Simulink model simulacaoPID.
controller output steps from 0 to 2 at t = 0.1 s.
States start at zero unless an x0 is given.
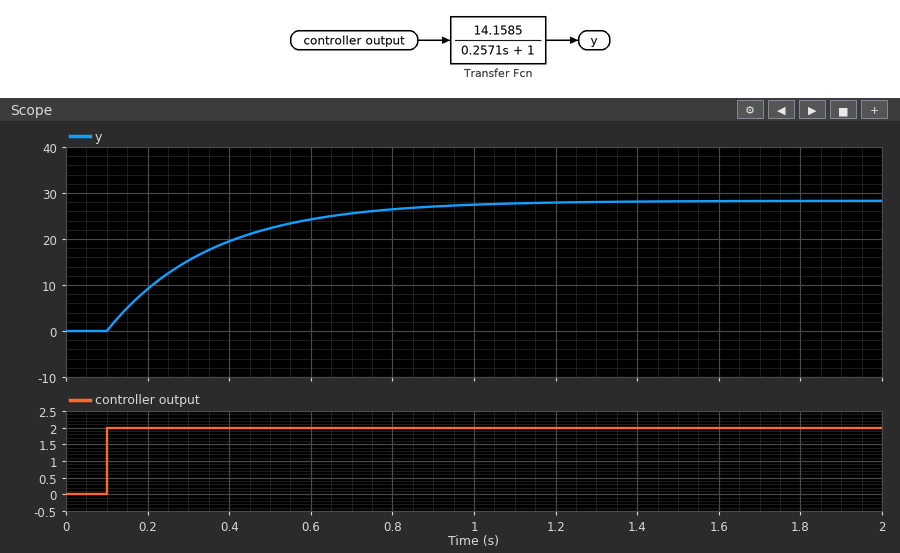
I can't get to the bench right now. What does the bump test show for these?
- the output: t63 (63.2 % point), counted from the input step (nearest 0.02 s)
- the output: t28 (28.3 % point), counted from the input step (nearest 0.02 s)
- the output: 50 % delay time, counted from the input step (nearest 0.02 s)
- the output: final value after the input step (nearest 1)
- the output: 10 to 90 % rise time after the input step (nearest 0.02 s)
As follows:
0.26 s
0.08 s
0.18 s
28
0.56 s
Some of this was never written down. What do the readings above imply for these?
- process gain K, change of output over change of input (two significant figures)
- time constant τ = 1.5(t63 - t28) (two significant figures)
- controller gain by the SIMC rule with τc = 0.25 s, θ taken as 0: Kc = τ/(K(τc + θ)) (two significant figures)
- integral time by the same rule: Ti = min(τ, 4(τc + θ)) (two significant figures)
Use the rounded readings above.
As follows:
14
0.27 s
0.077
0.27 s
